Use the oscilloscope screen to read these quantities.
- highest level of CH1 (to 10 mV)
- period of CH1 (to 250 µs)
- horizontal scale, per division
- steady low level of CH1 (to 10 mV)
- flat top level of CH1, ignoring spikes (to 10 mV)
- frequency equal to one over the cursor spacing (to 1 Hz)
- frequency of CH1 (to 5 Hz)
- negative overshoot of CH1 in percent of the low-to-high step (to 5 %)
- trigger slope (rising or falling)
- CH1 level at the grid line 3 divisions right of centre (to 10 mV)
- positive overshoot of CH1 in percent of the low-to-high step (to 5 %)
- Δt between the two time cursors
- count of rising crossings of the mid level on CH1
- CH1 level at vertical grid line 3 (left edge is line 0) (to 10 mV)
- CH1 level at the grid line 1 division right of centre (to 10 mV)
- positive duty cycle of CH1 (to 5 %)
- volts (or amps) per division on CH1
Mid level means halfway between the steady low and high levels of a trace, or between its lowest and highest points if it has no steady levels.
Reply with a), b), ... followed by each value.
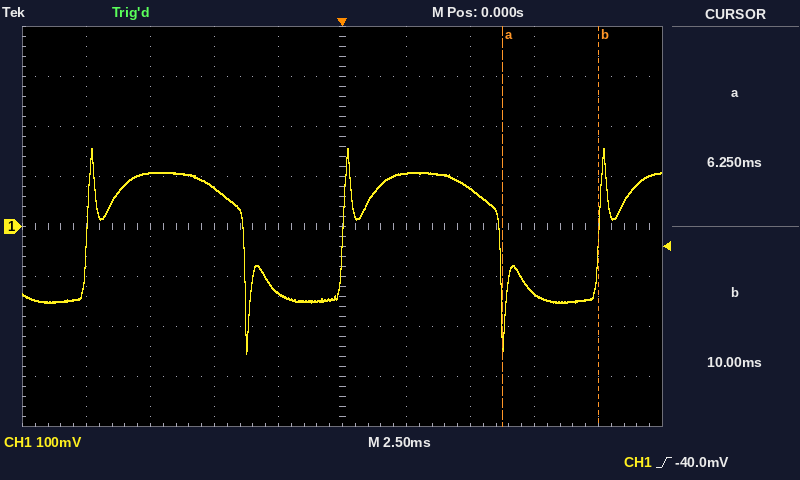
a) 160 mV
b) 10.00 ms
c) 2.5 ms
d) -150 mV
e) 110 mV
f) 267 Hz
g) 100 Hz
h) 40 %
i) rising
j) -130 mV
k) 20 %
l) 3.75 ms
m) 3
n) 80 mV
o) 110 mV
p) 60 %
q) 100 mV
